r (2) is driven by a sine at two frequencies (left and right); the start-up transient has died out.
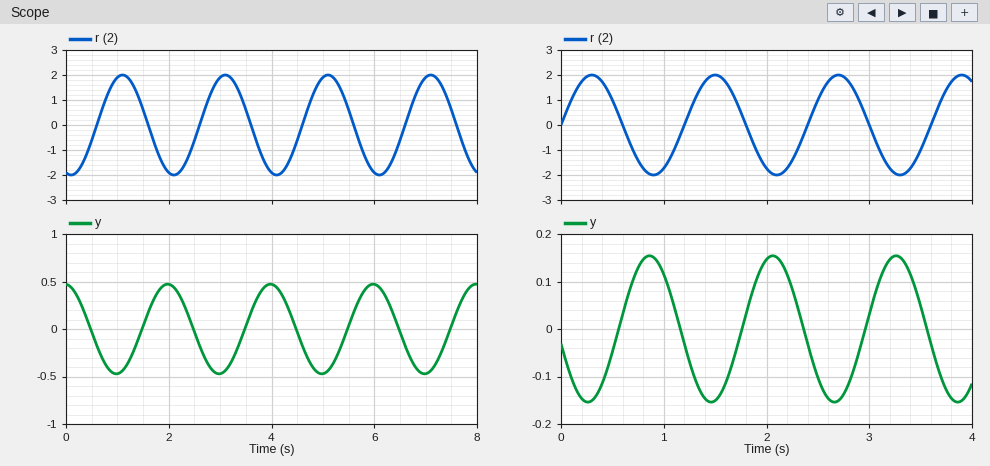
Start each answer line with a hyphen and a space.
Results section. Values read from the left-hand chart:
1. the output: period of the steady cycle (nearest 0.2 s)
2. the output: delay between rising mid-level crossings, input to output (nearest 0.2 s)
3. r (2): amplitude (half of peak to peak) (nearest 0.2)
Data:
- 2.0 s
- 0.8 s
- 2.0
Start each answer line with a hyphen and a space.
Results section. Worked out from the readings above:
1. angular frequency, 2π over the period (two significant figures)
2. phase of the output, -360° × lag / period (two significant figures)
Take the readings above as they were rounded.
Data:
- 3.1 rad/s
- -140°
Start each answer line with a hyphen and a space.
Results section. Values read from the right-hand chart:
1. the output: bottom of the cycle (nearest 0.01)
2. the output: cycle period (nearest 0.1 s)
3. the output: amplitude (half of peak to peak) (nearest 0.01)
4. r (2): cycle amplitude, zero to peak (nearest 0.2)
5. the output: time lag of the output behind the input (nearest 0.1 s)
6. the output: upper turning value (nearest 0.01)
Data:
- -0.15
- 1.2 s
- 0.15
- 2.0
- 0.6 s
- 0.15
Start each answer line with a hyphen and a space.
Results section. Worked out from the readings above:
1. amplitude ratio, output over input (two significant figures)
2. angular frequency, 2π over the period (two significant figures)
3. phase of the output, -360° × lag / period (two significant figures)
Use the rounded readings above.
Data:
- 0.075
- 5.2 rad/s
- -180°
